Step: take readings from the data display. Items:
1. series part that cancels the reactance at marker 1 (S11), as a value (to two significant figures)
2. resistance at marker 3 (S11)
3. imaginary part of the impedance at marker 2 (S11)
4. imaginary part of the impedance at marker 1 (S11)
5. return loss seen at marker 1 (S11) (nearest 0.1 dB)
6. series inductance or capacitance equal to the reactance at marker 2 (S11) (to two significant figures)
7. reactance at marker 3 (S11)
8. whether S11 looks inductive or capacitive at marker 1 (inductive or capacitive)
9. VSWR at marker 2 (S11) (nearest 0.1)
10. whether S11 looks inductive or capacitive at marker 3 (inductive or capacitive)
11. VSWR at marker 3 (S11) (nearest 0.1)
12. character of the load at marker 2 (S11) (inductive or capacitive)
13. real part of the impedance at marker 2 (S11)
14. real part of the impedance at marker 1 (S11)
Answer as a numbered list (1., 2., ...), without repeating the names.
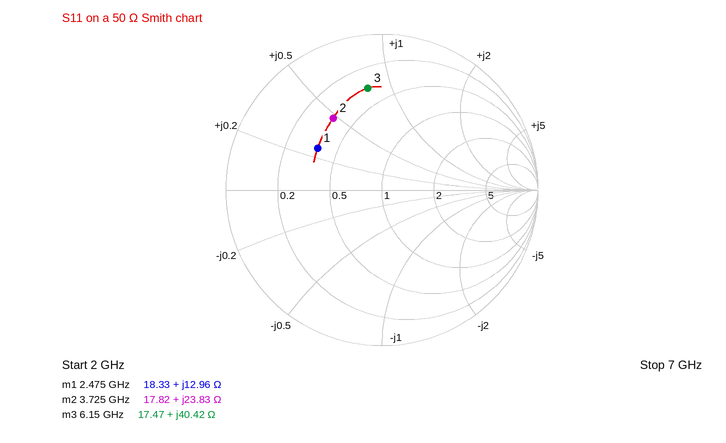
1. 5.0 pF
2. 17.47 Ω
3. +23.83 Ω
4. +12.96 Ω
5. 6.2 dB
6. 1.0 nH
7. +40.42 Ω
8. inductive
9. 3.5
10. inductive
11. 4.9
12. inductive
13. 17.82 Ω
14. 18.33 Ω
